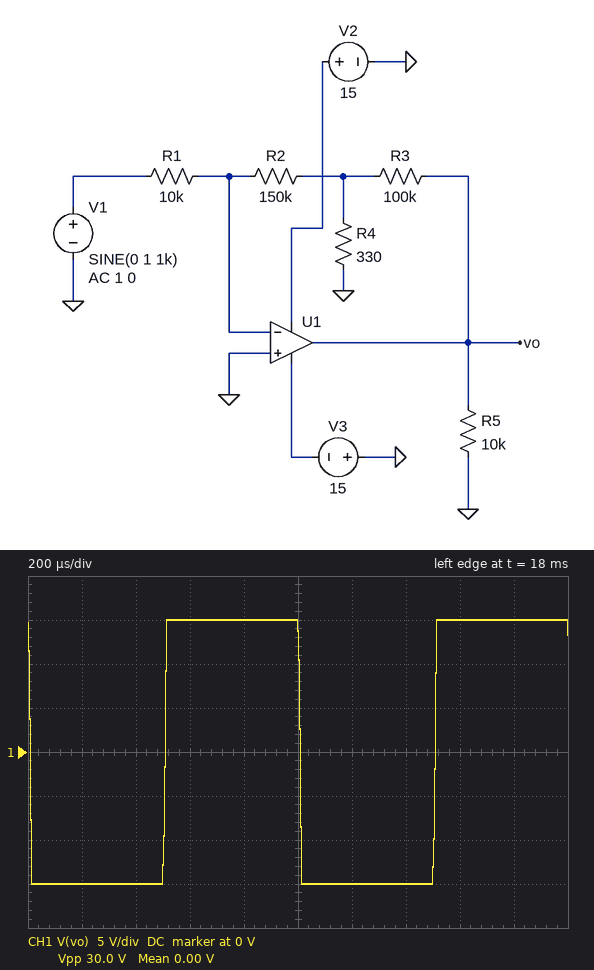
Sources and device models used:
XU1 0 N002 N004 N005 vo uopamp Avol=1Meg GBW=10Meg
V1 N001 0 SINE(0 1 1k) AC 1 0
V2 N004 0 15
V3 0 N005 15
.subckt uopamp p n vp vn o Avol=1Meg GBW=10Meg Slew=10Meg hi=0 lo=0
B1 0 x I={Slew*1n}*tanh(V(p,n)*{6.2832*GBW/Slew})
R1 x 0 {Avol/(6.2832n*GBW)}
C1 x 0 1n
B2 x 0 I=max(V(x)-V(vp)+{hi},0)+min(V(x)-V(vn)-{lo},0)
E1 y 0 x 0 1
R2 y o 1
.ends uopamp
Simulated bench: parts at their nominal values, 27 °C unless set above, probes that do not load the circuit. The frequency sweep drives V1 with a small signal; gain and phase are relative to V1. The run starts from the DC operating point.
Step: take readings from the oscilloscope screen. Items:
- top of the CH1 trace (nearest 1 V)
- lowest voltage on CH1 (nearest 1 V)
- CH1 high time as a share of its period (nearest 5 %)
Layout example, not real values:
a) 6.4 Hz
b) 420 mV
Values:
a) 15 V
b) -15 V
c) 50 %
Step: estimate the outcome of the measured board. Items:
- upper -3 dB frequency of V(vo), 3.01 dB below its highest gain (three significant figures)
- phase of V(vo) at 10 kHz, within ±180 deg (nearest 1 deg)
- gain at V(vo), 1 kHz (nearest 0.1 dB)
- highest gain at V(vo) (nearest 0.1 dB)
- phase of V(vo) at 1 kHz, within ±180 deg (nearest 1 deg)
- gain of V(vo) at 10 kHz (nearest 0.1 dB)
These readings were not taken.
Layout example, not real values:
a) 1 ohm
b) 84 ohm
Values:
a) 2.06 kHz
b) 102 deg
c) 72.2 dB
d) 73.2 dB
e) 154 deg
f) 59.3 dB
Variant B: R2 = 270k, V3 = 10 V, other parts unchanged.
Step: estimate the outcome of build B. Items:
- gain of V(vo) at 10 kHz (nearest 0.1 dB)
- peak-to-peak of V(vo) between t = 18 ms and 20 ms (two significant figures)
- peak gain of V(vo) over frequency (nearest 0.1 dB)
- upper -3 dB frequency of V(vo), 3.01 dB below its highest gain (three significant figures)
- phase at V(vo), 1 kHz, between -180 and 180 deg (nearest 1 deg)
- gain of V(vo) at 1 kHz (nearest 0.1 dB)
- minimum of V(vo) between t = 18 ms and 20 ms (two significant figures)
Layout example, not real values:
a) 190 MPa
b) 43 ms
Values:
a) 59.6 dB
b) 25 V
c) 78.2 dB
d) 1.18 kHz
e) 140 deg
f) 75.9 dB
g) -10 V
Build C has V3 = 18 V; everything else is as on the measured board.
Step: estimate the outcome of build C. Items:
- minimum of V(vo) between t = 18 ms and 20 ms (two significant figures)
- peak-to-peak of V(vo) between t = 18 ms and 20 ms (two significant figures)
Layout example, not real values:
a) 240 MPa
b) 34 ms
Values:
a) -18 V
b) 33 V
